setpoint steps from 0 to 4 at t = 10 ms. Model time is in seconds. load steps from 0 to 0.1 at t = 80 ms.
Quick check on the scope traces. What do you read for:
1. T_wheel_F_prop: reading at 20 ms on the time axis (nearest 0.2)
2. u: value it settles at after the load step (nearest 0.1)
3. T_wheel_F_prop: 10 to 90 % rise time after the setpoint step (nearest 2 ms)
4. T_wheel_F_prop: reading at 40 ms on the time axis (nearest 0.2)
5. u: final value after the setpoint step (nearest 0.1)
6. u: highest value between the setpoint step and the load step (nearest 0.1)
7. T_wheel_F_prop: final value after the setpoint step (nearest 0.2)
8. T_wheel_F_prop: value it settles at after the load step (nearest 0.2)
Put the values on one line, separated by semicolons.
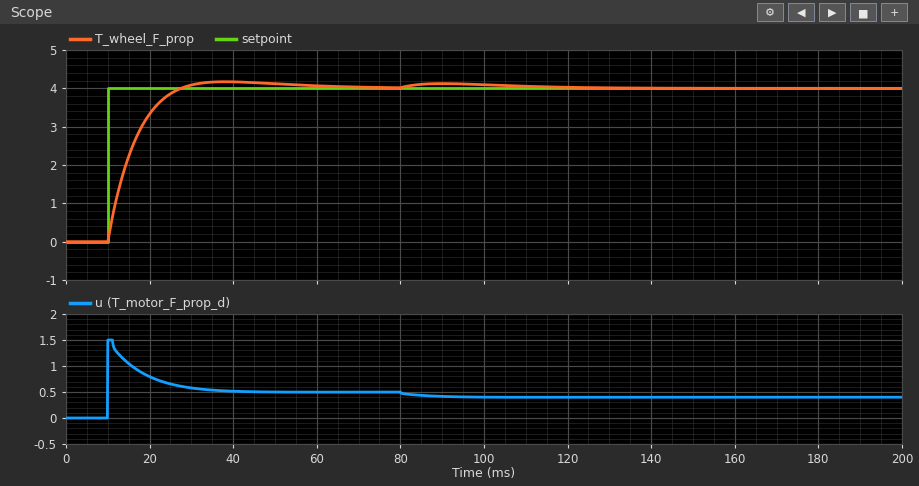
3.4; 0.4; 12 ms; 4.2; 0.5; 1.5; 4.0; 4.0
